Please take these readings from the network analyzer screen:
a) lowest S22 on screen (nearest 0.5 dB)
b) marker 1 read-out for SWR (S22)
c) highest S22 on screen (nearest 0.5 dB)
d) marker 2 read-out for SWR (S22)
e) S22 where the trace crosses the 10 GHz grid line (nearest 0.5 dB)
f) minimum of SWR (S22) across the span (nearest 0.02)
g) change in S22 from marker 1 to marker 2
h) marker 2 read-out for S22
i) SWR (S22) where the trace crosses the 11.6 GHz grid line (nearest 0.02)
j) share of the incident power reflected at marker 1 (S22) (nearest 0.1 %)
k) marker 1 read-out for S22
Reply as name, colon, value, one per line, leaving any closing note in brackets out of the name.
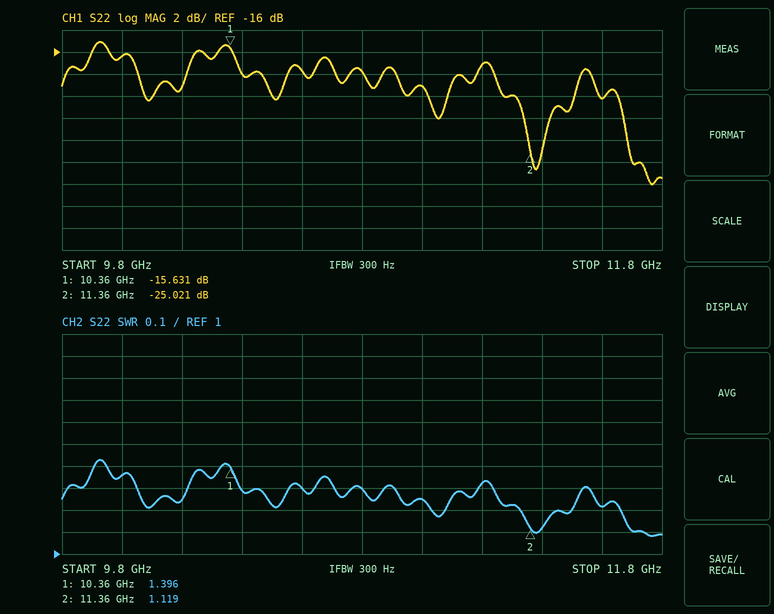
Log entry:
lowest S22 on screen: -28.0 dB
marker 1 read-out for SWR: 1.396
highest S22 on screen: -15.0 dB
marker 2 read-out for SWR: 1.119
S22 where the trace crosses the 10 GHz grid line: -16.5 dB
minimum of SWR (S22) across the span: 1.08
change in S22 from marker 1 to marker 2: -9.390 dB
marker 2 read-out for S22: -25.021 dB
SWR (S22) where the trace crosses the 11.6 GHz grid line: 1.22
share of the incident power reflected at marker 1 (S22): 2.7 %
marker 1 read-out for S22: -15.631 dB
